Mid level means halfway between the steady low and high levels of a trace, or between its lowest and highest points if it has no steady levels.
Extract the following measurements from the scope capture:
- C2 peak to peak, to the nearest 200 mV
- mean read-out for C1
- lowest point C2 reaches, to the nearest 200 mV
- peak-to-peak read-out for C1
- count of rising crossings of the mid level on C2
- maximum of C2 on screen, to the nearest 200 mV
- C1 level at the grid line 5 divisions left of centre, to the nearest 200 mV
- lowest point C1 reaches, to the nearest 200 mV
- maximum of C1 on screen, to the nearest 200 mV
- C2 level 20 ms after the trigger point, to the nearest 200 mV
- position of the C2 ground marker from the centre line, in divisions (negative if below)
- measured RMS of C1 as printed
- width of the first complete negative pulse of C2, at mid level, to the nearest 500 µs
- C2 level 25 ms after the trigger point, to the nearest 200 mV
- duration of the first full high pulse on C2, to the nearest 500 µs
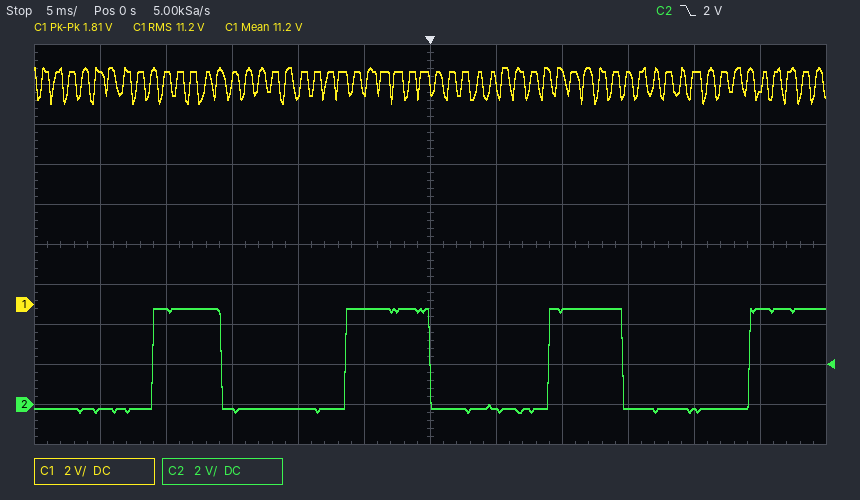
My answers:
5.2 V
11.2 V
-400 mV
1.81 V
4
4.8 V
11.6 V
10.0 V
11.8 V
-200 mV
-4.0 div
11.2 V
9.5 ms
4.8 V
5.0 ms
